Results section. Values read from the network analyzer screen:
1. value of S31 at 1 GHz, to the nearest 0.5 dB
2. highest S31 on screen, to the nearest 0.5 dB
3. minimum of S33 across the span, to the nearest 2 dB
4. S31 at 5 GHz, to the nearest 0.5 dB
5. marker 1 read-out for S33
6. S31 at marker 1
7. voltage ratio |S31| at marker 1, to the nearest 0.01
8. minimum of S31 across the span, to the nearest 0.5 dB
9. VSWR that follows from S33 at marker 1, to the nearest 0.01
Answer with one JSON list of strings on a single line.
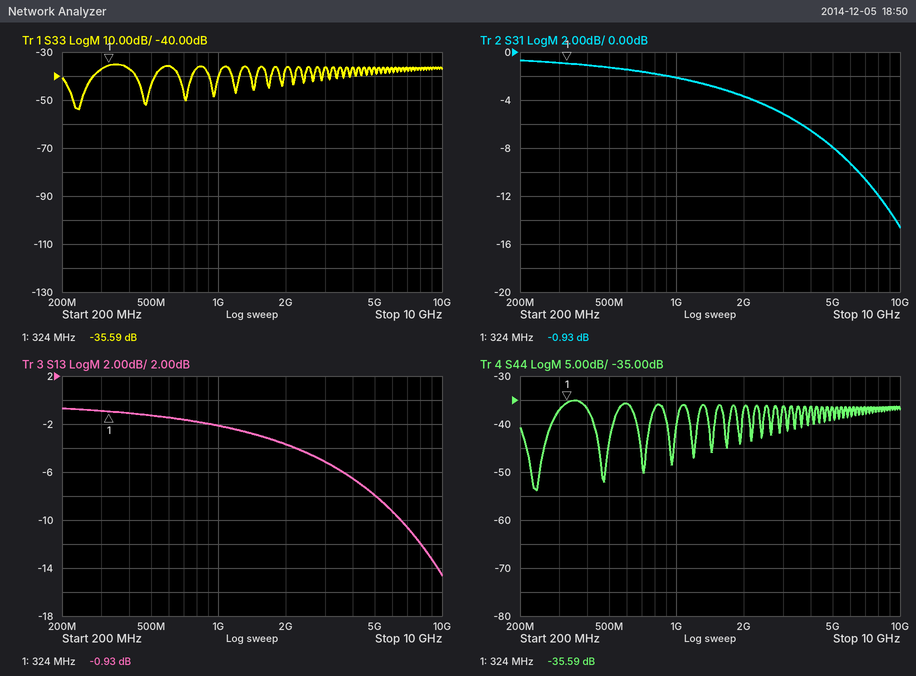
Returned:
["-2.0 dB", "-0.5 dB", "-54 dB", "-8.0 dB", "-35.59 dB", "-0.93 dB", "0.90", "-14.5 dB", "1.03"]
